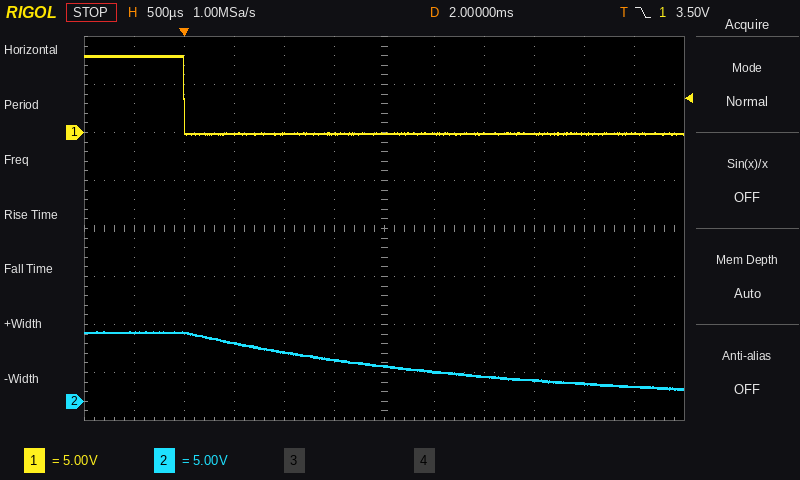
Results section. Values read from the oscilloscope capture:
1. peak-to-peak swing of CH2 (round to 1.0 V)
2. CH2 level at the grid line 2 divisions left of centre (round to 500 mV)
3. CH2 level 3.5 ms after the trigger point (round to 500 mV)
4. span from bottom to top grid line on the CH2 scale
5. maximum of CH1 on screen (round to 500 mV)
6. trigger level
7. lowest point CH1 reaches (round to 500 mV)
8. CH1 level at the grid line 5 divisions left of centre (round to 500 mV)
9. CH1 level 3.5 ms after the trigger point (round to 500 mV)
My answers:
6.0 V
5.0 V
2.0 V
40 V
8.0 V
3.50 V
0.0 V
8.0 V
0.0 V
